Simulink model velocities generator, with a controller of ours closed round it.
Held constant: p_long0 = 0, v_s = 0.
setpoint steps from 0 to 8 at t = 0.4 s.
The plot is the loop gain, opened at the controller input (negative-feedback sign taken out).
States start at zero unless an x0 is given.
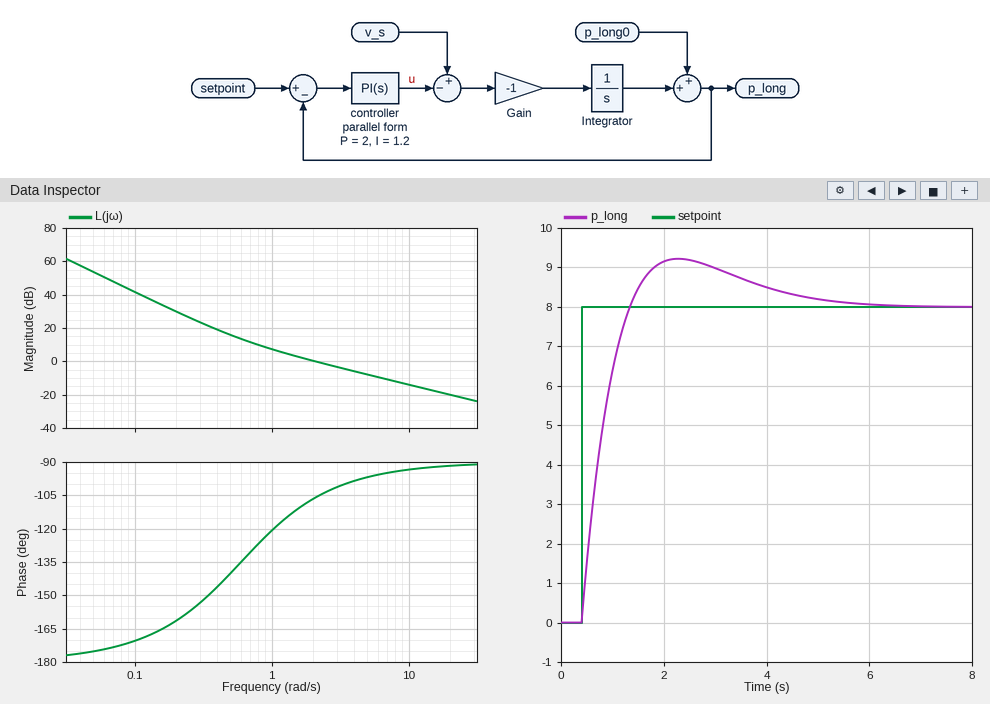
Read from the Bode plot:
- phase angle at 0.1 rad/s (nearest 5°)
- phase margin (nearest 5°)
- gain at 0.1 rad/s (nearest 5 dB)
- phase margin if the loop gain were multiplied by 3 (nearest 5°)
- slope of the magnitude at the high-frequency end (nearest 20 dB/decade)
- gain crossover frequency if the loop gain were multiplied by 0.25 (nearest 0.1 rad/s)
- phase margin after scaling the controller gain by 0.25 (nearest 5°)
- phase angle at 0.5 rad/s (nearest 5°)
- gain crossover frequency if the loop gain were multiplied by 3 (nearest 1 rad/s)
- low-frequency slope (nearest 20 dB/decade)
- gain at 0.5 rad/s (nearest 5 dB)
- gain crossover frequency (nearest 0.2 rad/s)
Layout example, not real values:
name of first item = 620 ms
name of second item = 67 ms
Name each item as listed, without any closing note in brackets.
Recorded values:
phase angle at 0.1 rad/s = -170°
phase margin = 75°
gain at 0.1 rad/s = 40 dB
phase margin if the loop gain were multiplied by 3 = 85°
slope of the magnitude at the high-frequency end = -20 dB/decade
gain crossover frequency if the loop gain were multiplied by 0.25 = 0.7 rad/s
phase margin after scaling the controller gain by 0.25 = 50°
phase angle at 0.5 rad/s = -140°
gain crossover frequency if the loop gain were multiplied by 3 = 6 rad/s
low-frequency slope = -40 dB/decade
gain at 0.5 rad/s = 15 dB
gain crossover frequency = 2.0 rad/s
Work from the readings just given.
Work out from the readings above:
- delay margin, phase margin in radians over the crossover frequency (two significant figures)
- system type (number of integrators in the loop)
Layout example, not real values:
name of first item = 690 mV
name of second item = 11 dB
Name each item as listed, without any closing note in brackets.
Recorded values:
delay margin, phase margin in radians over the crossover frequency = 0.65 s
system type = 2
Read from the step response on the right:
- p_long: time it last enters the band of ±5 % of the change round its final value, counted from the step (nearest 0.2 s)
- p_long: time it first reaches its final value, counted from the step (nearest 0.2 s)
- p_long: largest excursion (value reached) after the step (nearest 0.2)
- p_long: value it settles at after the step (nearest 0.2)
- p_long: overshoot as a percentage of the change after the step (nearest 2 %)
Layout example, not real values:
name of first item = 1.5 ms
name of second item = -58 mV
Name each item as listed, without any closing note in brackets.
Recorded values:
p_long: time it last enters the band of ±5 % of the change round its final value, counted from the step = 3.8 s
p_long: time it first reaches its final value, counted from the step = 1.0 s
p_long: largest excursion (value reached) after the step = 9.2
p_long: value it settles at after the step = 8.0
p_long: overshoot as a percentage of the change after the step = 16 %
